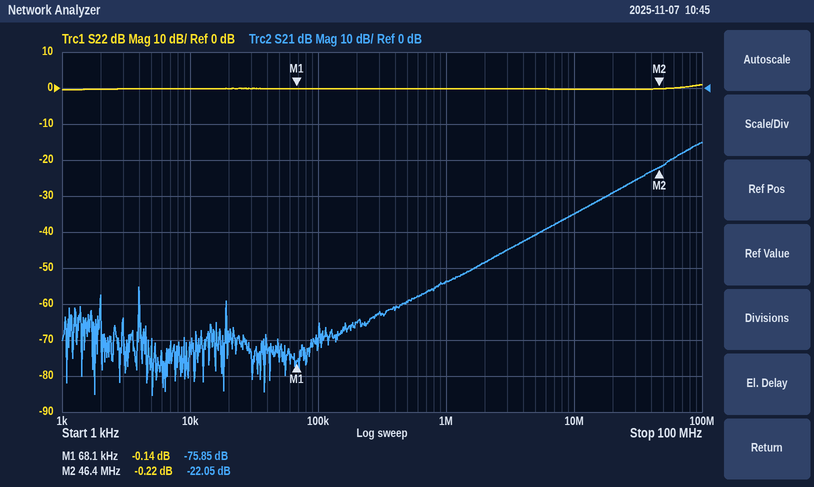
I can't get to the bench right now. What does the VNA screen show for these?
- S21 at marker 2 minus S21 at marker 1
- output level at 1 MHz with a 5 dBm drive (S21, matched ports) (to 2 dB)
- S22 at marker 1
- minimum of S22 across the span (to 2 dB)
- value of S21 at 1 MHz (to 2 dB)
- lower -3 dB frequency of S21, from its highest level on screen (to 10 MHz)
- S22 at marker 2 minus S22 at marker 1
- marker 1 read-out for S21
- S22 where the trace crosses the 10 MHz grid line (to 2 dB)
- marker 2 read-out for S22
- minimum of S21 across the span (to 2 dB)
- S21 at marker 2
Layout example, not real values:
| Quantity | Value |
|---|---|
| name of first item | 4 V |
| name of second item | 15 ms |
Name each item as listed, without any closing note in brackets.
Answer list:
| Quantity | Value |
|---|---|
| S21 at marker 2 minus S21 at marker 1 | 53.80 dB |
| output level at 1 MHz with a 5 dBm drive (S21, matched ports) | -48 dBm |
| S22 at marker 1 | -0.14 dB |
| minimum of S22 across the span | 0 dB |
| value of S21 at 1 MHz | -54 dB |
| lower -3 dB frequency of S21, from its highest level on screen | 70 MHz |
| S22 at marker 2 minus S22 at marker 1 | -0.08 dB |
| marker 1 read-out for S21 | -75.85 dB |
| S22 where the trace crosses the 10 MHz grid line | 0 dB |
| marker 2 read-out for S22 | -0.22 dB |
| minimum of S21 across the span | -86 dB |
| S21 at marker 2 | -22.05 dB |
